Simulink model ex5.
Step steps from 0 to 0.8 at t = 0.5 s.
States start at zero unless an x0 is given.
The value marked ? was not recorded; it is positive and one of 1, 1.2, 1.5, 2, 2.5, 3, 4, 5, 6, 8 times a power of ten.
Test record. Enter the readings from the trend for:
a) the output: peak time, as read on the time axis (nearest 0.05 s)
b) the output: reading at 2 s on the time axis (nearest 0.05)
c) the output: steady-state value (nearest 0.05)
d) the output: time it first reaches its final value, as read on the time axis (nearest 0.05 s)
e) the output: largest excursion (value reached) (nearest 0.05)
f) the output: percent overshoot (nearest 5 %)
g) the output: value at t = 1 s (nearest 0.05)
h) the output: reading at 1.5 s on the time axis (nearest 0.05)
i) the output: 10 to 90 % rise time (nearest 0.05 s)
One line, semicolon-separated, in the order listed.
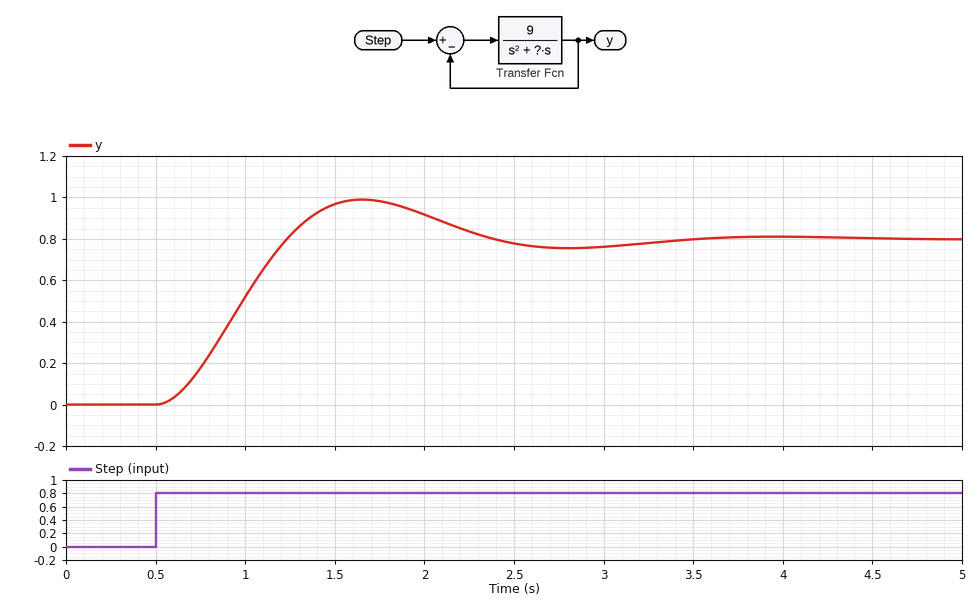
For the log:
1.65 s; 0.90; 0.80; 1.25 s; 1.00; 25 %; 0.50; 0.95; 0.50 s
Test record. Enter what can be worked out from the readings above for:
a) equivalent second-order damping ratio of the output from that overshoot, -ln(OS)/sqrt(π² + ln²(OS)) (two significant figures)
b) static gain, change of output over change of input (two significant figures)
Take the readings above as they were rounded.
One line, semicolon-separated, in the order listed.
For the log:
0.40; 1.0
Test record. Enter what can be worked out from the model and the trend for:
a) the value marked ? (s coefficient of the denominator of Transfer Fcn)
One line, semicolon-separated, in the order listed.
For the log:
2.5
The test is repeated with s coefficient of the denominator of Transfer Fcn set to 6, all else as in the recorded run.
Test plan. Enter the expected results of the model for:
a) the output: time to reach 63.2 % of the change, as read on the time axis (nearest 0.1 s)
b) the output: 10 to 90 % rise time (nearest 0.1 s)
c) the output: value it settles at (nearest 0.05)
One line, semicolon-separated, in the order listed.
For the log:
1.2 s; 1.1 s; 0.80
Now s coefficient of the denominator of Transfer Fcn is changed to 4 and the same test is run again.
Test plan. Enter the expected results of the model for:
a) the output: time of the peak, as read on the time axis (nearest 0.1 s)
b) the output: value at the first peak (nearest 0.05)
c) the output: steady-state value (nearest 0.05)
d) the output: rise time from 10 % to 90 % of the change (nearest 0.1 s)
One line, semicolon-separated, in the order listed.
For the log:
1.9 s; 0.85; 0.80; 0.7 s
